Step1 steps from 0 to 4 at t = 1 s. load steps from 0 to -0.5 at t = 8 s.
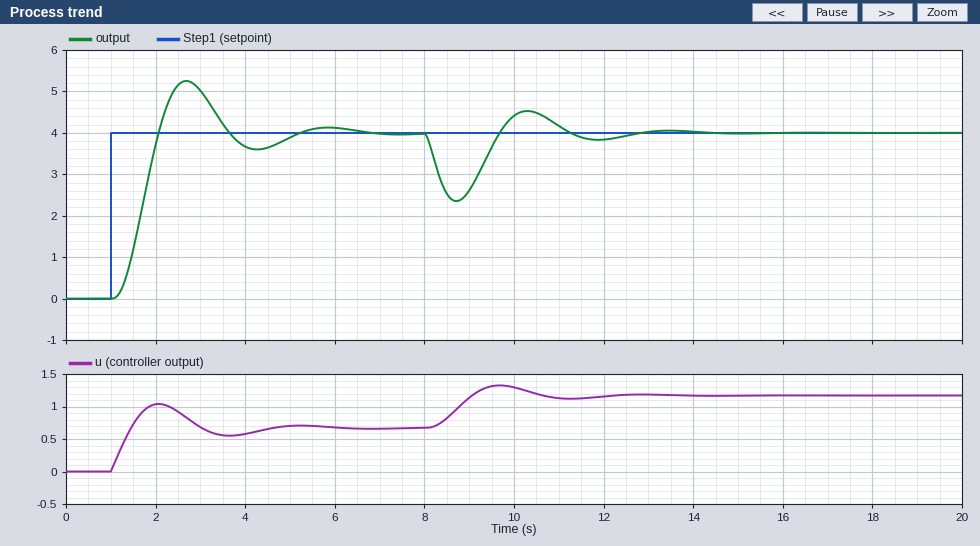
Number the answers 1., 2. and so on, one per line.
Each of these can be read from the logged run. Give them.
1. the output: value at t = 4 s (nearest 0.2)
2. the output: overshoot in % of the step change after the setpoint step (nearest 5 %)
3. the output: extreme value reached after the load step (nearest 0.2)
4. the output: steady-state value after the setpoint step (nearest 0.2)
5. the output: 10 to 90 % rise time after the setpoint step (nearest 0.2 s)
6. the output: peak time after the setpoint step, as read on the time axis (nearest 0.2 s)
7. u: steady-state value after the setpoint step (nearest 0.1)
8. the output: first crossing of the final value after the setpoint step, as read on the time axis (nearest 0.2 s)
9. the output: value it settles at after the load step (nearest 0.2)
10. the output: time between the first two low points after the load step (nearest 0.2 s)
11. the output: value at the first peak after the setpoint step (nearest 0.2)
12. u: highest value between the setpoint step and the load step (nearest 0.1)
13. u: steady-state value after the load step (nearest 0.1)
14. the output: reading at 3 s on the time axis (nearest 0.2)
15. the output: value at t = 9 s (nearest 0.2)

1. 3.6
2. 30 %
3. 2.4
4. 4.0
5. 0.6 s
6. 2.6 s
7. 0.7
8. 2.0 s
9. 4.0
10. 3.2 s
11. 5.2
12. 1.0
13. 1.2
14. 5.0
15. 2.6
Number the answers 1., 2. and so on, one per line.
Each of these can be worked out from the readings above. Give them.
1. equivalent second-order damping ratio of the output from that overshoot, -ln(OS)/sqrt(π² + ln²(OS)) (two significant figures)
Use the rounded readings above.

1. 0.36
